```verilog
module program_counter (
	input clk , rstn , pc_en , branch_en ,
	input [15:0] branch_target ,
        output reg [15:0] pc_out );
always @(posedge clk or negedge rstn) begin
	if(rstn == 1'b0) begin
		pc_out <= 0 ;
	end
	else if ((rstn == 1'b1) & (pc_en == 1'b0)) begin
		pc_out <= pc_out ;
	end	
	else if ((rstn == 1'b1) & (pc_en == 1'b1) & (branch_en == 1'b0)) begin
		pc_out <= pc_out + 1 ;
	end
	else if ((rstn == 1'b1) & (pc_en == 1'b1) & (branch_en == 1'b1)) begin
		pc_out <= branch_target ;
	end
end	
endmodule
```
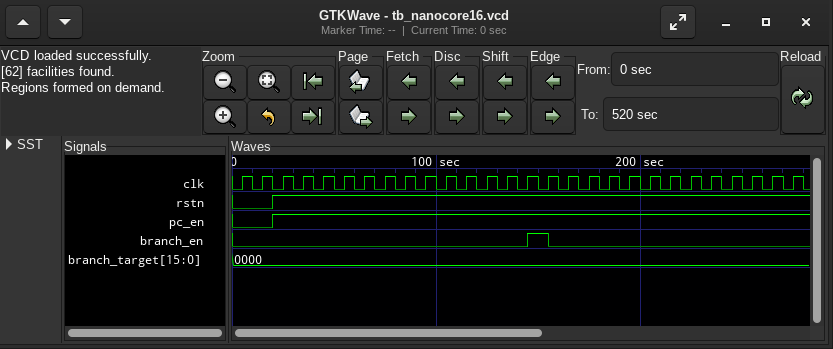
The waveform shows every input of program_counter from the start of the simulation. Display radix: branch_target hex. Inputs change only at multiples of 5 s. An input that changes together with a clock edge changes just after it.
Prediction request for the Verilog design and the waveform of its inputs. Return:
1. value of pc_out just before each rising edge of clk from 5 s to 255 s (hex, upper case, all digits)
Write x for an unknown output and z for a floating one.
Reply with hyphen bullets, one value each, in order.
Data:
- 0000, 0000, 0000, 0001, 0002, 0003, 0004, 0005, 0006, 0007, 0008, 0009, 000A, 000B, 000C, 000D, 0000, 0001, 0002, 0003, 0004, 0005, 0006, 0007, 0008, 0009
